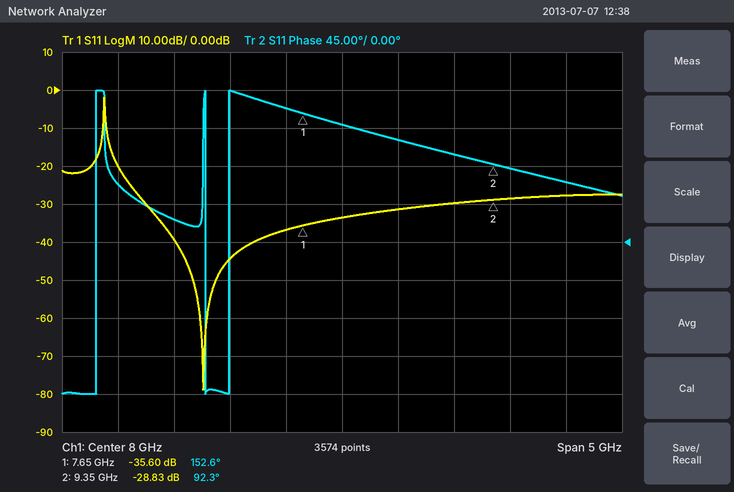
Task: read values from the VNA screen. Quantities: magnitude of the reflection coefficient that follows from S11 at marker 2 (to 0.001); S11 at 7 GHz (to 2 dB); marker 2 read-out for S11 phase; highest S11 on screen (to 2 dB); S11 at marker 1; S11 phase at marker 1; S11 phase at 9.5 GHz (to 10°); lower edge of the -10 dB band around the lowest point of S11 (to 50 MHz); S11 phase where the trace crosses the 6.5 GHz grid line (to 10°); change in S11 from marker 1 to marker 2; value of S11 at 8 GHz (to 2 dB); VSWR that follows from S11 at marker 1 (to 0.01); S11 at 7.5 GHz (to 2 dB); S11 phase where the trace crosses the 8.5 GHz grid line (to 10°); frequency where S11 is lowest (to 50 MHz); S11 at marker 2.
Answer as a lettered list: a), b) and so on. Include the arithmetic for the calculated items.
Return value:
a) 10^(-28.83/20) ≈ 0.036
b) -44 dB
c) 92.3°
d) -2 dB
e) -35.60 dB
f) 152.6°
g) 90°
h) 5.90 GHz
i) 30°
j) -28.83 − (-35.6) = 6.77 dB
k) -34 dB
l) (1 + 0.0166)/(1 − 0.0166) ≈ 1.03
m) -36 dB
n) 120°
o) 6.75 GHz
p) -28.83 dB
